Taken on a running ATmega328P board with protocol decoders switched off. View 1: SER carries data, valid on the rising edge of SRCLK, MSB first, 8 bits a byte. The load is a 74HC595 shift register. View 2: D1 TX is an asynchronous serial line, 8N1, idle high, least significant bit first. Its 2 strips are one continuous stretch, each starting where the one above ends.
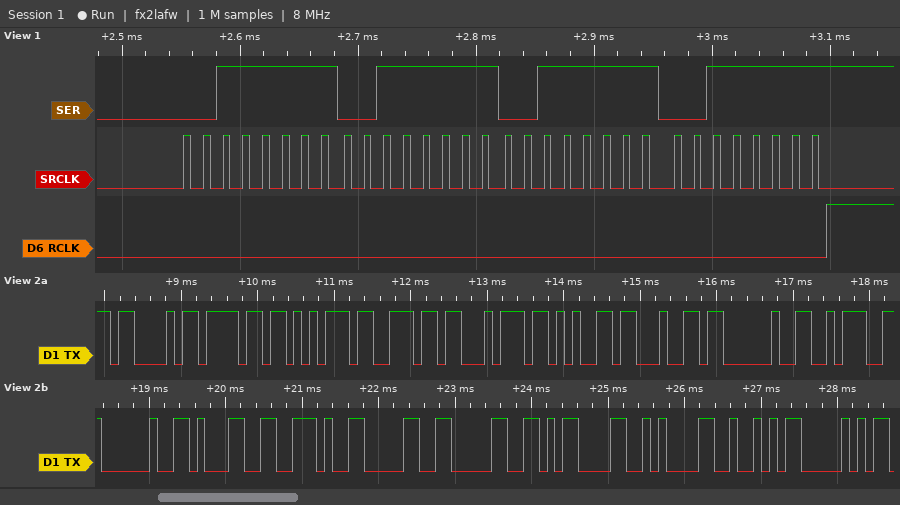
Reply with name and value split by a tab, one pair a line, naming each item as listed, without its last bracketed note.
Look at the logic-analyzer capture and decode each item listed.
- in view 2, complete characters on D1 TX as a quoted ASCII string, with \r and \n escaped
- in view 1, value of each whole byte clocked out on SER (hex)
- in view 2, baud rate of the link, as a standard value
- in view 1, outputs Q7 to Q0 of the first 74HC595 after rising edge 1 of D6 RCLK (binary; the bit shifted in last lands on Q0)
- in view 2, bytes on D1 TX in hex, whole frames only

in view 2, complete characters on D1 TX as a quoted ASCII string, with \r and \n escaped	"Counted : 1.00\r\nRP"
in view 1, value of each whole byte clocked out on SER	3F 3F 3F 3F
in view 2, baud rate of the link, as a standard value	9600 baud
in view 1, outputs Q7 to Q0 of the first 74HC595 after rising edge 1 of D6 RCLK	00111111
in view 2, bytes on D1 TX in hex, whole frames only	0x43 0x6F 0x75 0x6E 0x74 0x65 0x64 0x20 0x3A 0x20 0x31 0x2E 0x30 0x30 0x0D 0x0A 0x52 0x50
